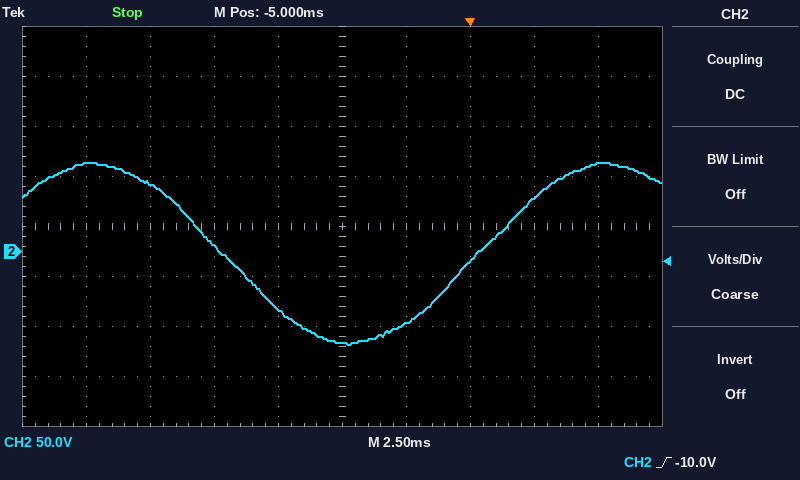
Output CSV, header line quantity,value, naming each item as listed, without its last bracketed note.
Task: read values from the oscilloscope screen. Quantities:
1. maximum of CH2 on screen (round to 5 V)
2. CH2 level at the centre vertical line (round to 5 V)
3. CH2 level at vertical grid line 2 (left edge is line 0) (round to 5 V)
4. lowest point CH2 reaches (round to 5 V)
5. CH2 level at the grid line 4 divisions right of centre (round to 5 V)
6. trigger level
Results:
quantity,value
maximum of CH2 on screen,90 V
CH2 level at the centre vertical line,-90 V
CH2 level at vertical grid line 2 (left edge is line 0),70 V
lowest point CH2 reaches,-95 V
CH2 level at the grid line 4 divisions right of centre,90 V
trigger level,-10.0 V
